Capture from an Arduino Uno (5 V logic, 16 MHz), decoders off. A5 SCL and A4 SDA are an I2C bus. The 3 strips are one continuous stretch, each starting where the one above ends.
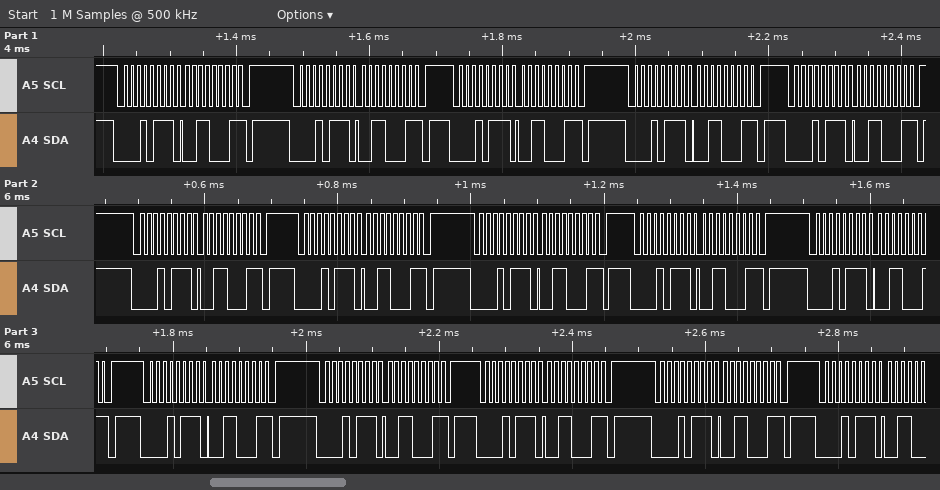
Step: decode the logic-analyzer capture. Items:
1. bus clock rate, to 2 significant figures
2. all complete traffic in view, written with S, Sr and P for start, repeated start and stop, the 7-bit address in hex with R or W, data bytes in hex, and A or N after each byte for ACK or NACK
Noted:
100 kHz
S 0BR A 31 N P S 0BR A 31 N P S 0BR A 31 N P S 0BR A 31 N P S 0BR A 31 N P S 0BR A 31 N P S 0BR A 31 N P S 0BR A 31 N P S 0BR A 31 N P S 0BR A 31 N P S 0BR A 31 N P S 0BR A 31 N P S 0BR A 31 N P S 0BR A 31 N P S 0BR A
